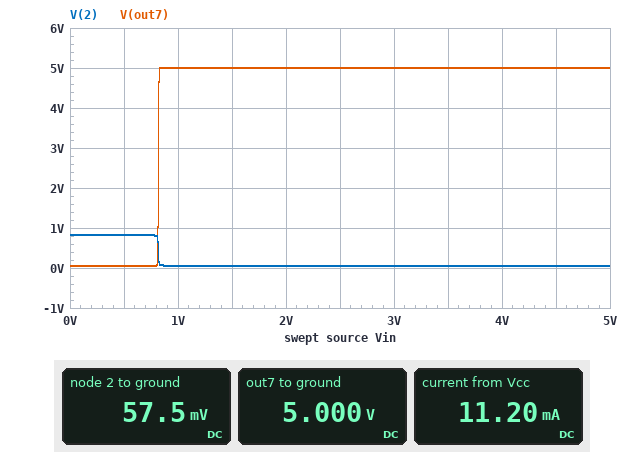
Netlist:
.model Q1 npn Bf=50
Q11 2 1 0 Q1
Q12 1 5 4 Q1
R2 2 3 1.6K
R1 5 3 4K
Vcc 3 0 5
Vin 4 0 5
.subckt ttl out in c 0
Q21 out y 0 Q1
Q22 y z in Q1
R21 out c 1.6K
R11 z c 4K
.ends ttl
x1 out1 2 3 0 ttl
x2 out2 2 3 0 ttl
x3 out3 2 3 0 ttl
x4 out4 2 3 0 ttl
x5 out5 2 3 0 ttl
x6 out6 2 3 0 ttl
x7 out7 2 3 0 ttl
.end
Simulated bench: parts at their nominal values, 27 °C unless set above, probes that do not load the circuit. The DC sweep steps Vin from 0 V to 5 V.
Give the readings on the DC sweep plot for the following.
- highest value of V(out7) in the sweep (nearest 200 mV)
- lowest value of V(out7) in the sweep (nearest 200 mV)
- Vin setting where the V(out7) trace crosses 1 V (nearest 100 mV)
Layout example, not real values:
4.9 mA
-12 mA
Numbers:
5.0 V
0 V
800 mV
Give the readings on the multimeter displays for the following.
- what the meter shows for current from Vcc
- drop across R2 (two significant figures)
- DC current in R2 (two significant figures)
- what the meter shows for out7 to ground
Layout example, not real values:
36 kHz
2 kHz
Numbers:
11.20 mA
4.9 V
3.1 mA
5.000 V
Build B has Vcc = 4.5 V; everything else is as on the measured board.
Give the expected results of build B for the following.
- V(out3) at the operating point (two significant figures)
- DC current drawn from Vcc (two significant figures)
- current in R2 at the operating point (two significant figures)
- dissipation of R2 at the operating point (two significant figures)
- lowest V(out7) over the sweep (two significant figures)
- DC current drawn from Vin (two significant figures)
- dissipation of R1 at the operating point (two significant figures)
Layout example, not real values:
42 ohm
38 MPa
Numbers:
4.5 V
9.9 mA
2.8 mA
12 mW
41 mV
720 µA
2.1 mW
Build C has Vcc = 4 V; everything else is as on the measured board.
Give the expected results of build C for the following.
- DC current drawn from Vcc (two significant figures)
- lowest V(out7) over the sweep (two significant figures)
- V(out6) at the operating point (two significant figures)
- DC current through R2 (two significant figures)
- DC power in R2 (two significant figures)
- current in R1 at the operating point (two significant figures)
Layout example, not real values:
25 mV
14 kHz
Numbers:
8.6 mA
42 mV
4.0 V
2.5 mA
9.7 mW
600 µA
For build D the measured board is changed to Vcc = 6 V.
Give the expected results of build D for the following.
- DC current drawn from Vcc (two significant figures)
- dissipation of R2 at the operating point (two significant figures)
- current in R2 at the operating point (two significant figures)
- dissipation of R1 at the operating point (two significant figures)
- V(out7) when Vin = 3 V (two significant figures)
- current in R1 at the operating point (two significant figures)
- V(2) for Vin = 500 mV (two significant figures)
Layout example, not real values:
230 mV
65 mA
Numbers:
14 mA
22 mW
3.7 mA
4.8 mW
6.0 V
1.1 mA
840 mV
